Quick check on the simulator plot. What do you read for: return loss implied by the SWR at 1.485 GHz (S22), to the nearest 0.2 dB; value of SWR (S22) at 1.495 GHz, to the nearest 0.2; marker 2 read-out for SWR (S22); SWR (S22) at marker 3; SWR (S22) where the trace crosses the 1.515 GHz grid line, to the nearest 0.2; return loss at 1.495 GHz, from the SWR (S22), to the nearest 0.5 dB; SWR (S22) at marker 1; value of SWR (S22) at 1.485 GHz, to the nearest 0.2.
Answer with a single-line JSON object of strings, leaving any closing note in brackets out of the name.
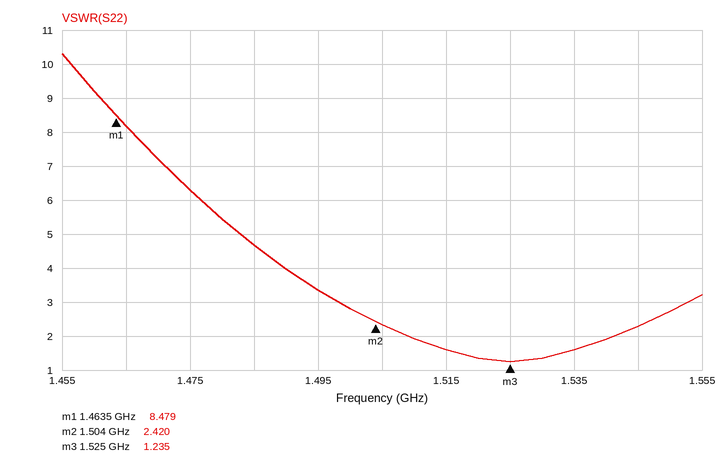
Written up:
{"return loss implied by the SWR at 1.485 GHz (S22), to the nearest 0.2 dB": "3.8 dB", "value of SWR (S22) at 1.495 GHz, to the nearest 0.2": "3.4", "marker 2 read-out for SWR": "2.420", "SWR (S22) at marker 3": "1.235", "SWR (S22) where the trace crosses the 1.515 GHz grid line, to the nearest 0.2": "1.6", "return loss at 1.495 GHz, from the SWR (S22), to the nearest 0.5 dB": "5.5 dB", "SWR (S22) at marker 1": "8.479", "value of SWR (S22) at 1.485 GHz, to the nearest 0.2": "4.6"}
